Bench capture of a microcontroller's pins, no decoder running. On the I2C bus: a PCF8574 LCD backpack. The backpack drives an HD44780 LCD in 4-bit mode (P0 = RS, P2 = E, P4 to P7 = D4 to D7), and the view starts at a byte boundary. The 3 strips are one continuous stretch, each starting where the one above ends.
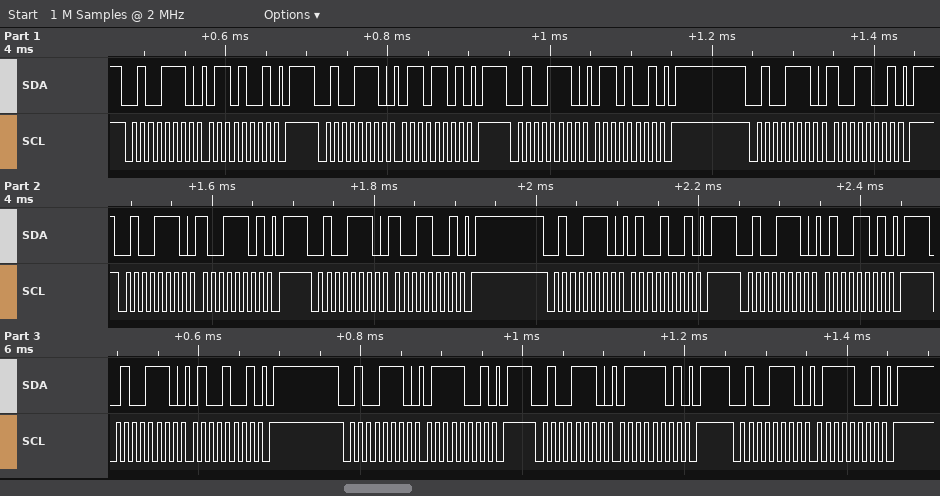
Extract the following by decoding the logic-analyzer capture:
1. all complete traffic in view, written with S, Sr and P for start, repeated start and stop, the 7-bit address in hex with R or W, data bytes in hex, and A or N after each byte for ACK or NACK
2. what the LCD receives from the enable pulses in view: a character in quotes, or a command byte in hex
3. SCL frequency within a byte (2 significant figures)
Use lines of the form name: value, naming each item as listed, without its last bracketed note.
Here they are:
all complete traffic in view, written with S, Sr and P for start, repeated start and stop, the 7-bit address in hex with R or W, data bytes in hex, and A or N after each byte for ACK or NACK: S 27W A 69 A P S 27W A 6D A P S 27W A 69 A P S 27W A 99 A P S 27W A 9D A P S 27W A 99 A P S 27W A 49 A P S 27W A 4D A P S 27W A 49 A P S 27W A 79 A P S 27W A 7D A P S 27W A 79 A P
what the LCD receives from the enable pulses in view: a character in quotes, or a command byte in hex: 'i' 'G'
SCL frequency within a byte: 100 kHz
